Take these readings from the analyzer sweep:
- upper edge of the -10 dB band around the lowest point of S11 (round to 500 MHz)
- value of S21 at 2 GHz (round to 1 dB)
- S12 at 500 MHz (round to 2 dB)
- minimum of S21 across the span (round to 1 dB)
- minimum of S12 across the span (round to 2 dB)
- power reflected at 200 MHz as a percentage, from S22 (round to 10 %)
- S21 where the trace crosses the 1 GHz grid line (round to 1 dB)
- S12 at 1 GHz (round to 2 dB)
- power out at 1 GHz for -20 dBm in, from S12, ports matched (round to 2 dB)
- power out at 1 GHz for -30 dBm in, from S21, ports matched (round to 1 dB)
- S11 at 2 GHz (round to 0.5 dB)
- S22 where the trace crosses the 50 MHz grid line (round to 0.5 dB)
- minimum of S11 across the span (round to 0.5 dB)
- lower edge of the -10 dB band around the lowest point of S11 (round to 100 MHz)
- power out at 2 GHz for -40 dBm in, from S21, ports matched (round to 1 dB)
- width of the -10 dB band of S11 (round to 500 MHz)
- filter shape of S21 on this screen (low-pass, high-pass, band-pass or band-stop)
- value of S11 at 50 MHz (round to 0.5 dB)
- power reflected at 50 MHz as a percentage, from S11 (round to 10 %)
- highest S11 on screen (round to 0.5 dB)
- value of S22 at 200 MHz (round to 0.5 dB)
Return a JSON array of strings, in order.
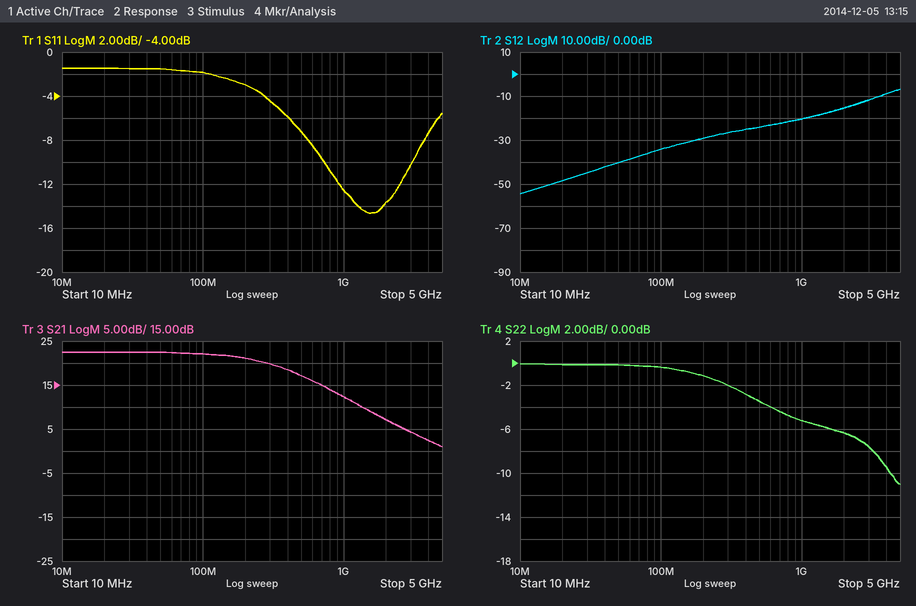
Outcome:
["3.0 GHz", "7 dB", "-24 dB", "1 dB", "-54 dB", "80 %", "12 dB", "-20 dB", "-40 dBm", "-18 dBm", "-13.5 dB", "0.0 dB", "-14.5 dB", "700 MHz", "-33 dBm", "2.5 GHz", "low-pass", "-1.5 dB", "70 %", "-1.5 dB", "-1.0 dB"]
